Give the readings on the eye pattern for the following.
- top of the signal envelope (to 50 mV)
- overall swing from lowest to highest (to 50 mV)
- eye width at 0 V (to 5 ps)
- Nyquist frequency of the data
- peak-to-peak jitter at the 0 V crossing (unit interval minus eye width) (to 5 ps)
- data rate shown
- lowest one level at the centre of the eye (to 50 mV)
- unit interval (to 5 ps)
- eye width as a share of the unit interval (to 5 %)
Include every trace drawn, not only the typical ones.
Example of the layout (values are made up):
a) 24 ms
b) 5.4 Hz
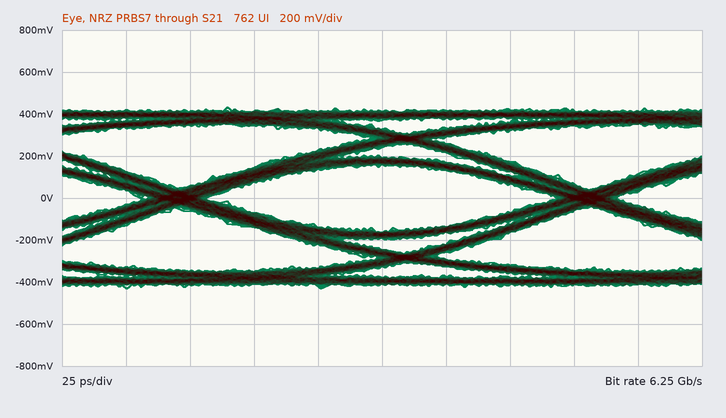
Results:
a) 450 mV
b) 850 mV
c) 135 ps
d) 3.125 GHz
e) 25 ps
f) 6.25 Gb/s
g) 150 mV
h) 160 ps
i) 85 %
